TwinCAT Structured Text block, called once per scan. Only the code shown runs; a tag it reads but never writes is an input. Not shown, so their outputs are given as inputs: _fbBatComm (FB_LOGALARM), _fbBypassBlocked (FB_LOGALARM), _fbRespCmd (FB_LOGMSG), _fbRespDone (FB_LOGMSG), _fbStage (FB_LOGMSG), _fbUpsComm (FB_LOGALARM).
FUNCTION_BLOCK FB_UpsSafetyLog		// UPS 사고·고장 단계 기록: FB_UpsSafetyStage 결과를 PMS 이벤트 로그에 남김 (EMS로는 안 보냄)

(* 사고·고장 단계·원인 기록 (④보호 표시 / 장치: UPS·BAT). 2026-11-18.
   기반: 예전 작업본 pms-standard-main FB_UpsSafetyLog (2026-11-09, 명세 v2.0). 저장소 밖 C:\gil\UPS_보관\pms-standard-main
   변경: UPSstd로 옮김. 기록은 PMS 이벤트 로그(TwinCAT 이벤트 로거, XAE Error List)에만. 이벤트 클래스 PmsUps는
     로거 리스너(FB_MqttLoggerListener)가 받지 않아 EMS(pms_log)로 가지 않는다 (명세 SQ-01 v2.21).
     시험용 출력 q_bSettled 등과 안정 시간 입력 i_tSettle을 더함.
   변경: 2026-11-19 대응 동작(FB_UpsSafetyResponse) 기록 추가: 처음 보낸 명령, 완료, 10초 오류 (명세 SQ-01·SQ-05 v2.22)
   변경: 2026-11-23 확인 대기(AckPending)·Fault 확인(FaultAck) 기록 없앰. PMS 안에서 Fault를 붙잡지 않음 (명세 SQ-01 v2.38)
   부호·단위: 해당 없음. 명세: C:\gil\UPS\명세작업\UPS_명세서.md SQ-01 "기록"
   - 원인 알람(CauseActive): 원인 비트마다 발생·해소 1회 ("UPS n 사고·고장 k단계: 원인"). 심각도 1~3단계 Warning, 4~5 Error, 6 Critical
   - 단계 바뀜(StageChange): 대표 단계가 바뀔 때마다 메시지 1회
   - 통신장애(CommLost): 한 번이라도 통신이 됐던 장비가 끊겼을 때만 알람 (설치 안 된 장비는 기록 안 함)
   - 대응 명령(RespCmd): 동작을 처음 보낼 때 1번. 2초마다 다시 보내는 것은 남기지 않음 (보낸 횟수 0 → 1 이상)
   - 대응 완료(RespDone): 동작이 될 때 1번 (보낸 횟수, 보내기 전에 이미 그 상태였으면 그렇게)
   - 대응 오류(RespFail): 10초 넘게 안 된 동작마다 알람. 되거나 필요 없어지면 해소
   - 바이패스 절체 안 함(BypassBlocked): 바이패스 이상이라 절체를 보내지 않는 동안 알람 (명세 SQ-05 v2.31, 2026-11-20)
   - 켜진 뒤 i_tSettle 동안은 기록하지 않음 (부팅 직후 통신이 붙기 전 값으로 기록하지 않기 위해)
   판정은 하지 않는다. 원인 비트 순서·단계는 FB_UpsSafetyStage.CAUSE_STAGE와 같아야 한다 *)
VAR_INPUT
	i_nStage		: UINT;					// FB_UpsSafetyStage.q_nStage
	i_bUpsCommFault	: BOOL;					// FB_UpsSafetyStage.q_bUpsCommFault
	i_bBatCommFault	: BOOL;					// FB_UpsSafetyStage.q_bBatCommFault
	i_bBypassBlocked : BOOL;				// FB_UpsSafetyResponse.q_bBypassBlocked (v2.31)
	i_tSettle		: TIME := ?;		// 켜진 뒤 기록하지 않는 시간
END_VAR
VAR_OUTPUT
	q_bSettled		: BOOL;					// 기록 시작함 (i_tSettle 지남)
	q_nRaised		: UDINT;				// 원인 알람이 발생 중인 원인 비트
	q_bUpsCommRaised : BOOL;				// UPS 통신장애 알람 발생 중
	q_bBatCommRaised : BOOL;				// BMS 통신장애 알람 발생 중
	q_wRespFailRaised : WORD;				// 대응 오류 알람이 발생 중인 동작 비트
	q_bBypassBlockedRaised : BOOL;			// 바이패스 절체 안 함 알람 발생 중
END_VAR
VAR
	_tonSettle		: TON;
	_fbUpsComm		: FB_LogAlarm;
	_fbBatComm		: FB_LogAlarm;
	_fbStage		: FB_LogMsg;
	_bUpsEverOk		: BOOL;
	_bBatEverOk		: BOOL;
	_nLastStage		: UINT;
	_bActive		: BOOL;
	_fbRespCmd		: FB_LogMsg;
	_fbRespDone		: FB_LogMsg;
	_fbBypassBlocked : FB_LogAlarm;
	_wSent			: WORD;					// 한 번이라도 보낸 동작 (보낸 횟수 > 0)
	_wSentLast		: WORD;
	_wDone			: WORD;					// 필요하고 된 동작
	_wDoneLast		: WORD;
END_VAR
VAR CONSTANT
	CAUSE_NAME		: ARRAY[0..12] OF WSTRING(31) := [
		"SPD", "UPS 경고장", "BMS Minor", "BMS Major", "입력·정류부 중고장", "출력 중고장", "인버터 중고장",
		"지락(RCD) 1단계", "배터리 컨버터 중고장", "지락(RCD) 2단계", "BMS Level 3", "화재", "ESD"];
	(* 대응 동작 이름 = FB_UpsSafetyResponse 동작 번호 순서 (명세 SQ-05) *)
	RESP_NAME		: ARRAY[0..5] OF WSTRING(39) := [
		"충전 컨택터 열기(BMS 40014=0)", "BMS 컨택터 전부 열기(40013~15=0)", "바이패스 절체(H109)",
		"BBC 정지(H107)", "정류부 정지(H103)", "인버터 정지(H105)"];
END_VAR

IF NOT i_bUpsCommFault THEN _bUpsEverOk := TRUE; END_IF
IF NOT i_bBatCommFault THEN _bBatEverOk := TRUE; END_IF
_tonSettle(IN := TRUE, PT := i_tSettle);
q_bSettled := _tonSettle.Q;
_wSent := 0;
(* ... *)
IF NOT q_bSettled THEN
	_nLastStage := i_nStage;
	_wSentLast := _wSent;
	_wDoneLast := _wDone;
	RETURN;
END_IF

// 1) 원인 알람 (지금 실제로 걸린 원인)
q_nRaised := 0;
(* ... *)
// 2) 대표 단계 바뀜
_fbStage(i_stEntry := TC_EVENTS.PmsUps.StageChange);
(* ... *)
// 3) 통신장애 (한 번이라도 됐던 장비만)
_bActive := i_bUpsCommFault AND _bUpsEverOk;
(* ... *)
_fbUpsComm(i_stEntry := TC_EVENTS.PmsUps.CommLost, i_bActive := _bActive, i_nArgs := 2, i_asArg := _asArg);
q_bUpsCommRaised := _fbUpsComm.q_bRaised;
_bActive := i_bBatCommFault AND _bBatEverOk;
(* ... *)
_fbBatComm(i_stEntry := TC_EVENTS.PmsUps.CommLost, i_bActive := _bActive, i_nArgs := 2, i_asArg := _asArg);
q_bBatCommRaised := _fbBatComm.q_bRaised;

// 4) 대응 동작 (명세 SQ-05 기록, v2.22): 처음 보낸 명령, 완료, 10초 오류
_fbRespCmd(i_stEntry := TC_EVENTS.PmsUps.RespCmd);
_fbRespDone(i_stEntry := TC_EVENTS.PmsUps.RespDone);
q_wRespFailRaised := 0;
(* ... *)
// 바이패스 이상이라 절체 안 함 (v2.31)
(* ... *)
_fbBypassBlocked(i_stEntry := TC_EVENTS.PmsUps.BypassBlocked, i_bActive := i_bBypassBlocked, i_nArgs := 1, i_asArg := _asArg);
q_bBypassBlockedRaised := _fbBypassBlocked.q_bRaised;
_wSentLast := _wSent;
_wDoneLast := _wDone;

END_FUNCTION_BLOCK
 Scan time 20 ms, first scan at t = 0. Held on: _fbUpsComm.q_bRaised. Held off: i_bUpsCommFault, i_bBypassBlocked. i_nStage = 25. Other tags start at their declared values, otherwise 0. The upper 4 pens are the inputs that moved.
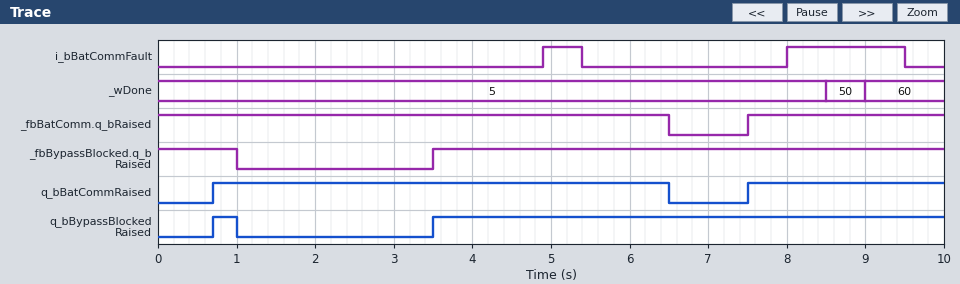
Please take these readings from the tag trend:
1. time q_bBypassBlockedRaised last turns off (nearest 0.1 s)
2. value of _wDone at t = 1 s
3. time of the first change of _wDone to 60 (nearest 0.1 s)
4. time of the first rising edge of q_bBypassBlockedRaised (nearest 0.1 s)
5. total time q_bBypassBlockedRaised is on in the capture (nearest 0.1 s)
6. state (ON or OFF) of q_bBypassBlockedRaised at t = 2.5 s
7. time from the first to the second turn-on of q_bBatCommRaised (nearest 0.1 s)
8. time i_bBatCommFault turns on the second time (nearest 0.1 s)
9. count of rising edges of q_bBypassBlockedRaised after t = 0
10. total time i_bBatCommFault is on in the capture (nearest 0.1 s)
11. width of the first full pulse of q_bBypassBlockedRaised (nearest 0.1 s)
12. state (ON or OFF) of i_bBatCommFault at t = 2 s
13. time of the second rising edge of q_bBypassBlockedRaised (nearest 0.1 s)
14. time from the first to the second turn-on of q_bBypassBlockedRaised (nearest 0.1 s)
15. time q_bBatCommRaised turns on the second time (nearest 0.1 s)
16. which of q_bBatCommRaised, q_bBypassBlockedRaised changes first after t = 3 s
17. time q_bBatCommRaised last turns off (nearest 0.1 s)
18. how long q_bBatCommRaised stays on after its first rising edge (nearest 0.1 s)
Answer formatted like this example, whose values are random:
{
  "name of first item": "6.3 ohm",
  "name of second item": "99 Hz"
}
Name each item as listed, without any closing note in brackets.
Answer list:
{
  "time q_bBypassBlockedRaised last turns off": "1.0 s",
  "value of _wDone at t = 1 s": "5",
  "time of the first change of _wDone to 60": "9.0 s",
  "time of the first rising edge of q_bBypassBlockedRaised": "0.7 s",
  "total time q_bBypassBlockedRaised is on in the capture": "6.8 s",
  "state (ON or OFF) of q_bBypassBlockedRaised at t = 2.5 s": "OFF",
  "time from the first to the second turn-on of q_bBatCommRaised": "6.8 s",
  "time i_bBatCommFault turns on the second time": "8.0 s",
  "count of rising edges of q_bBypassBlockedRaised after t = 0": "2",
  "total time i_bBatCommFault is on in the capture": "2.0 s",
  "width of the first full pulse of q_bBypassBlockedRaised": "0.3 s",
  "state (ON or OFF) of i_bBatCommFault at t = 2 s": "OFF",
  "time of the second rising edge of q_bBypassBlockedRaised": "3.5 s",
  "time from the first to the second turn-on of q_bBypassBlockedRaised": "2.8 s",
  "time q_bBatCommRaised turns on the second time": "7.5 s",
  "which of q_bBatCommRaised, q_bBypassBlockedRaised changes first after t = 3 s": "q_bBypassBlockedRaised",
  "time q_bBatCommRaised last turns off": "6.5 s",
  "how long q_bBatCommRaised stays on after its first rising edge": "5.8 s"
}
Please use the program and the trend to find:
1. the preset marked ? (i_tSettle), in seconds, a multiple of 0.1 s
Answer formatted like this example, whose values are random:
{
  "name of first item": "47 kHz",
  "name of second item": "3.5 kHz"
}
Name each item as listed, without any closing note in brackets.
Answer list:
{
  "the preset marked ? (i_tSettle), in seconds, a multiple of 0.1 s": "0.7 s"
}
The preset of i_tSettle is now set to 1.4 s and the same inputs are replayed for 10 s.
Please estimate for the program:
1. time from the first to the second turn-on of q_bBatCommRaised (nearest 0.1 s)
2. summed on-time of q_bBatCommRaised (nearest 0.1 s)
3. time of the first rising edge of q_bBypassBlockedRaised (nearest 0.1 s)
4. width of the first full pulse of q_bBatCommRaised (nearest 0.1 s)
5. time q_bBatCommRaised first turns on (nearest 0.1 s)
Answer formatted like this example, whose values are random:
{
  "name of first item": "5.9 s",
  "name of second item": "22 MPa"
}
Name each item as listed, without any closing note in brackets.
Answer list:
{
  "time from the first to the second turn-on of q_bBatCommRaised": "6.1 s",
  "summed on-time of q_bBatCommRaised": "7.6 s",
  "time of the first rising edge of q_bBypassBlockedRaised": "3.5 s",
  "width of the first full pulse of q_bBatCommRaised": "5.1 s",
  "time q_bBatCommRaised first turns on": "1.4 s"
}
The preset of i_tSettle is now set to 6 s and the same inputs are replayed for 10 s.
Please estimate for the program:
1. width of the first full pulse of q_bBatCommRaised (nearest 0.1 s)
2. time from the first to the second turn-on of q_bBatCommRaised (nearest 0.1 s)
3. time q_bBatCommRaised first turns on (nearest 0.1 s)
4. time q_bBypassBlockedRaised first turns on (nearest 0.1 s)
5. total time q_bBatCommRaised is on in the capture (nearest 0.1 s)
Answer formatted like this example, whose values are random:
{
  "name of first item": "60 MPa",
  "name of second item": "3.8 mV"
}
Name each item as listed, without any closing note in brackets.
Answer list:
{
  "width of the first full pulse of q_bBatCommRaised": "0.5 s",
  "time from the first to the second turn-on of q_bBatCommRaised": "1.5 s",
  "time q_bBatCommRaised first turns on": "6.0 s",
  "time q_bBypassBlockedRaised first turns on": "6.0 s",
  "total time q_bBatCommRaised is on in the capture": "3.0 s"
}
